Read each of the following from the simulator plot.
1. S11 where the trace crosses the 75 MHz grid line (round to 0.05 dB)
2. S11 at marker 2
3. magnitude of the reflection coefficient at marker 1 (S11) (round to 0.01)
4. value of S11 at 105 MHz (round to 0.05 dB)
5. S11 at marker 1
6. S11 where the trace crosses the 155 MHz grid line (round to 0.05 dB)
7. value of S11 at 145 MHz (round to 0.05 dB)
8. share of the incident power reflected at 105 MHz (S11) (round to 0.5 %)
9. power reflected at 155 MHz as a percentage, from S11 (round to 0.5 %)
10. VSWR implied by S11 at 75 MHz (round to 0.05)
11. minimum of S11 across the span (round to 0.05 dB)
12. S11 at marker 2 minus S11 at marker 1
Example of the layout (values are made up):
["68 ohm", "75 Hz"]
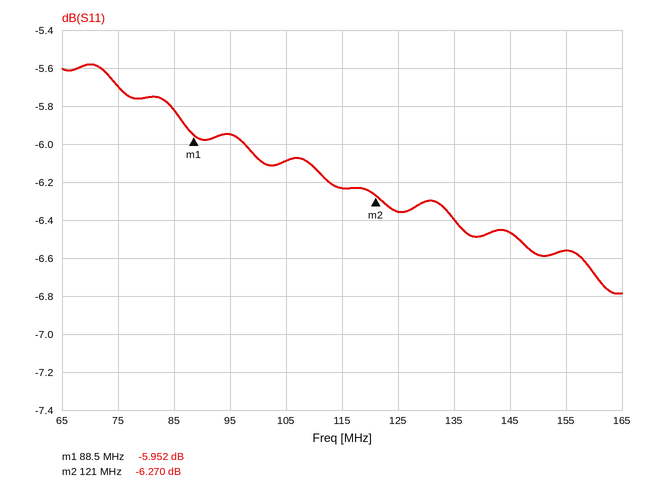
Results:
["-5.70 dB", "-6.270 dB", "0.50", "-6.10 dB", "-5.952 dB", "-6.55 dB", "-6.45 dB", "24.5 %", "22.0 %", "3.15", "-6.80 dB", "-0.318 dB"]
